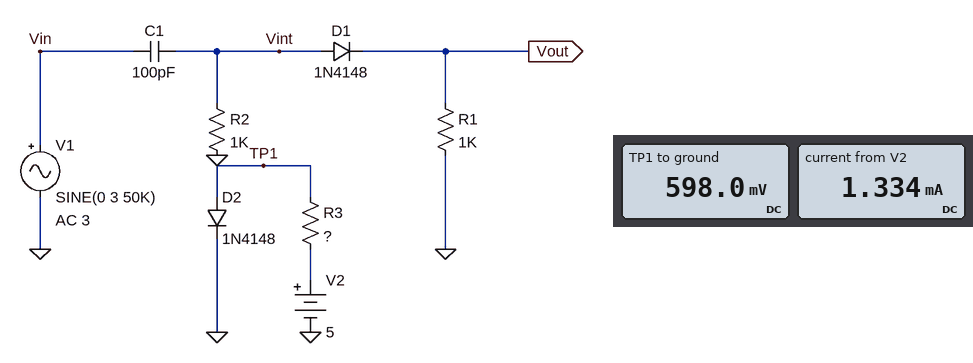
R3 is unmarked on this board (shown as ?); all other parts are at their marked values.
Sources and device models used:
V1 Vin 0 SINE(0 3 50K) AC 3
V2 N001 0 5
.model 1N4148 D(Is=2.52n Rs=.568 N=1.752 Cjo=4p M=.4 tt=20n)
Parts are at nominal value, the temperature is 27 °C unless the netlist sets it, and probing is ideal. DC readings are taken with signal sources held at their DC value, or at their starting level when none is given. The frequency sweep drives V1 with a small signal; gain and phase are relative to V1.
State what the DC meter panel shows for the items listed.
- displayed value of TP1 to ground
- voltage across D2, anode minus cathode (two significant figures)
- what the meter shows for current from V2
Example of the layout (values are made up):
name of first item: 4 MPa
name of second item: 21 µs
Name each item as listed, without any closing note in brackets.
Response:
displayed value of TP1 to ground: 598.0 mV
voltage across D2, anode minus cathode: 600 mV
what the meter shows for current from V2: 1.334 mA
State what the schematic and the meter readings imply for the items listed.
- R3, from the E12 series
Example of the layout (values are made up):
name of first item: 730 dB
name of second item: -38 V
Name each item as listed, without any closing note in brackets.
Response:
R3, from the E12 series: 3.3 kΩ
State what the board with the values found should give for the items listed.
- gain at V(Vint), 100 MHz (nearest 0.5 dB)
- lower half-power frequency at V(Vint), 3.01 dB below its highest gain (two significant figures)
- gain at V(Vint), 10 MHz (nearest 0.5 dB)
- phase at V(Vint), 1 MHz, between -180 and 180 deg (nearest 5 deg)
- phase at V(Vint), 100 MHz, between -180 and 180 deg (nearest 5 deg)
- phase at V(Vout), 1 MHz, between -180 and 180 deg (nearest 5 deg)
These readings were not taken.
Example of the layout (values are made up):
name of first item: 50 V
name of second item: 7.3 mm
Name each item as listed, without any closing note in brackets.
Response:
gain at V(Vint), 100 MHz: 0 dB
lower half-power frequency at V(Vint), 3.01 dB below its highest gain: 1.7 MHz
gain at V(Vint), 10 MHz: -0.5 dB
phase at V(Vint), 1 MHz, between -180 and 180 deg: 55 deg
phase at V(Vint), 100 MHz, between -180 and 180 deg: 0 deg
phase at V(Vout), 1 MHz, between -180 and 180 deg: 145 deg
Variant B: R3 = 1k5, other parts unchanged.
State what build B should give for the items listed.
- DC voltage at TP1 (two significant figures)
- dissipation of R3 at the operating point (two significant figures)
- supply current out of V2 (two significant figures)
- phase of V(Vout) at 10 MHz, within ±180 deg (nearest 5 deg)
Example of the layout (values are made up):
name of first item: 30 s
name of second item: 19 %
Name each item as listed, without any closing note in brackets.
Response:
DC voltage at TP1: 630 mV
dissipation of R3 at the operating point: 13 mW
supply current out of V2: 2.9 mA
phase of V(Vout) at 10 MHz, within ±180 deg: 85 deg
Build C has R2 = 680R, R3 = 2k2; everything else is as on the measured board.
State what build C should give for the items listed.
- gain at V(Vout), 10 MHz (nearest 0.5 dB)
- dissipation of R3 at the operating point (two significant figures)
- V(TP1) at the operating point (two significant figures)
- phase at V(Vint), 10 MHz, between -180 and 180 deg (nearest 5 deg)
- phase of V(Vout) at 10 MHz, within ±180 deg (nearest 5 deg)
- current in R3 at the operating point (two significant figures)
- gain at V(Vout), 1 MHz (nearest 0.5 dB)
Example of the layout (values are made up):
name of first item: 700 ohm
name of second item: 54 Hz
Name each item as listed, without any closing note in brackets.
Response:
gain at V(Vout), 10 MHz: -13.0 dB
dissipation of R3 at the operating point: 8.7 mW
V(TP1) at the operating point: 620 mV
phase at V(Vint), 10 MHz, between -180 and 180 deg: 15 deg
phase of V(Vout) at 10 MHz, within ±180 deg: 90 deg
current in R3 at the operating point: 2.0 mA
gain at V(Vout), 1 MHz: -40.0 dB
